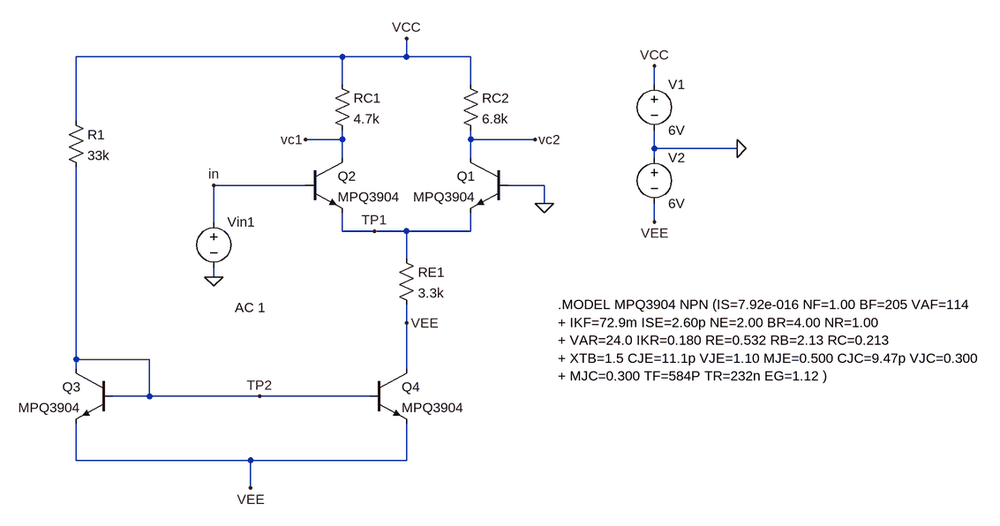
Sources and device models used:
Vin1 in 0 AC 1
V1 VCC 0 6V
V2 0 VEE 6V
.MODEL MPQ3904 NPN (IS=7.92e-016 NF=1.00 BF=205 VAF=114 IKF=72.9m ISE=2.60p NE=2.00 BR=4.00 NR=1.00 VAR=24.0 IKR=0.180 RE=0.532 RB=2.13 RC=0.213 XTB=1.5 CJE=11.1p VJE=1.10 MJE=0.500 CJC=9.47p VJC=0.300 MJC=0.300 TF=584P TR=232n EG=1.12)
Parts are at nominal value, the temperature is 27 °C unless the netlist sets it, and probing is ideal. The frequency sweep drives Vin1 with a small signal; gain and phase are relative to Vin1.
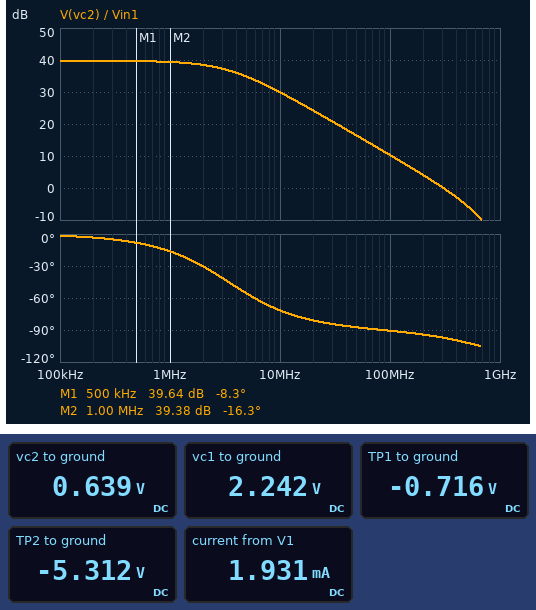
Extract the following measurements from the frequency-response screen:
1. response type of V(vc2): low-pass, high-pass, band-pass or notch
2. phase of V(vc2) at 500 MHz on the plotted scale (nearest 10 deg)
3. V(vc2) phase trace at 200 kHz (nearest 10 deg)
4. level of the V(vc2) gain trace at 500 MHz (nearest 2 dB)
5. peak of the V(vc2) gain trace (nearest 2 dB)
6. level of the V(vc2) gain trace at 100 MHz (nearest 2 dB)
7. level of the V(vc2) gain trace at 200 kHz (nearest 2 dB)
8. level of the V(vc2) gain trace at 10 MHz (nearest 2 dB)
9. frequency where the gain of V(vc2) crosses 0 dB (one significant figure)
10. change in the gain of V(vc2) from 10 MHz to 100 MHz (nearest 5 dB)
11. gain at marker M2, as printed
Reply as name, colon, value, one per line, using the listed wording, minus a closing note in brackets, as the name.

response type of V(vc2): low-pass, high-pass, band-pass or notch: low-pass
phase of V(vc2) at 500 MHz on the plotted scale: -100 deg
V(vc2) phase trace at 200 kHz: 0 deg
level of the V(vc2) gain trace at 500 MHz: -6 dB
peak of the V(vc2) gain trace: 40 dB
level of the V(vc2) gain trace at 100 MHz: 10 dB
level of the V(vc2) gain trace at 200 kHz: 40 dB
level of the V(vc2) gain trace at 10 MHz: 30 dB
frequency where the gain of V(vc2) crosses 0 dB: 300 MHz
change in the gain of V(vc2) from 10 MHz to 100 MHz: -20 dB
gain at marker M2, as printed: 39.38 dB
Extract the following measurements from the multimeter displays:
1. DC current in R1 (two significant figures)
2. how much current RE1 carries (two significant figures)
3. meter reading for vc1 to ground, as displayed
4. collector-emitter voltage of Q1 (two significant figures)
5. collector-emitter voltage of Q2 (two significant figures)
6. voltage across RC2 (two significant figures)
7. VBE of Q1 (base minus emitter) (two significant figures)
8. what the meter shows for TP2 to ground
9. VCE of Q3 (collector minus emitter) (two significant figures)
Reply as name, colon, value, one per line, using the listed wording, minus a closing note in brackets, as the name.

DC current in R1: 340 µA
how much current RE1 carries: 1.6 mA
meter reading for vc1 to ground, as displayed: 2.242 V
collector-emitter voltage of Q1: 1.4 V
collector-emitter voltage of Q2: 3.0 V
voltage across RC2: 5.4 V
VBE of Q1 (base minus emitter): 720 mV
what the meter shows for TP2 to ground: -5.312 V
VCE of Q3 (collector minus emitter): 690 mV
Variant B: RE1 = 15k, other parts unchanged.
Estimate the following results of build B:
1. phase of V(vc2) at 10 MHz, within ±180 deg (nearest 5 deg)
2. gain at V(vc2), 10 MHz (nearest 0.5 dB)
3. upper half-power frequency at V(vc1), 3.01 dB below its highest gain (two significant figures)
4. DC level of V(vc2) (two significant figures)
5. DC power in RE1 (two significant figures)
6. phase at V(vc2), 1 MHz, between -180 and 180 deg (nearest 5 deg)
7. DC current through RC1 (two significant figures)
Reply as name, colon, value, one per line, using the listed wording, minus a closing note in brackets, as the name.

phase of V(vc2) at 10 MHz, within ±180 deg: -60 deg
gain at V(vc2), 10 MHz: 21.0 dB
upper half-power frequency at V(vc1), 3.01 dB below its highest gain: 8.5 MHz
DC level of V(vc2): 4.8 V
DC power in RE1: 1.9 mW
phase at V(vc2), 1 MHz, between -180 and 180 deg: -10 deg
DC current through RC1: 180 µA
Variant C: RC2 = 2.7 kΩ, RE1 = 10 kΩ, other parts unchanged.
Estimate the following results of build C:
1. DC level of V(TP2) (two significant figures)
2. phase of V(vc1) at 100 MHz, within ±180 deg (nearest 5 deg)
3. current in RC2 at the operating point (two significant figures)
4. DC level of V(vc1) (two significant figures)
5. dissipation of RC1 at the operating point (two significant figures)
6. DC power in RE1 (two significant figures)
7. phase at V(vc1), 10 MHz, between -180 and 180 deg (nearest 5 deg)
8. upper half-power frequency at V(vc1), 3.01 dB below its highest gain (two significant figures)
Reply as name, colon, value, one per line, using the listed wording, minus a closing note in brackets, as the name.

DC level of V(TP2): -5.3 V
phase of V(vc1) at 100 MHz, within ±180 deg: 65 deg
current in RC2 at the operating point: 260 µA
DC level of V(vc1): 4.8 V
dissipation of RC1 at the operating point: 320 µW
DC power in RE1: 2.8 mW
phase at V(vc1), 10 MHz, between -180 and 180 deg: 125 deg
upper half-power frequency at V(vc1), 3.01 dB below its highest gain: 8.3 MHz
